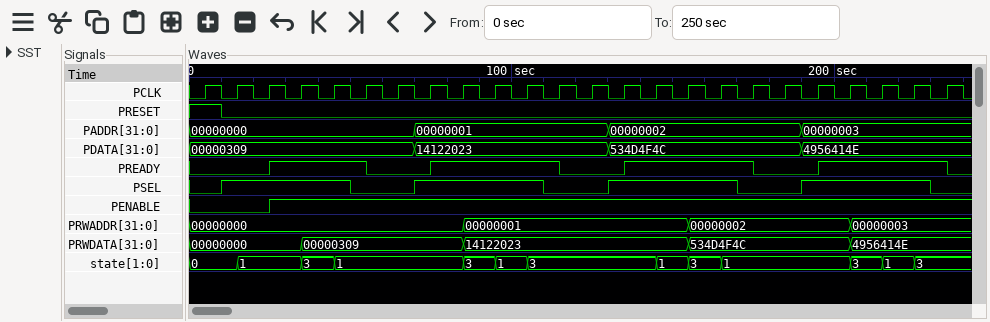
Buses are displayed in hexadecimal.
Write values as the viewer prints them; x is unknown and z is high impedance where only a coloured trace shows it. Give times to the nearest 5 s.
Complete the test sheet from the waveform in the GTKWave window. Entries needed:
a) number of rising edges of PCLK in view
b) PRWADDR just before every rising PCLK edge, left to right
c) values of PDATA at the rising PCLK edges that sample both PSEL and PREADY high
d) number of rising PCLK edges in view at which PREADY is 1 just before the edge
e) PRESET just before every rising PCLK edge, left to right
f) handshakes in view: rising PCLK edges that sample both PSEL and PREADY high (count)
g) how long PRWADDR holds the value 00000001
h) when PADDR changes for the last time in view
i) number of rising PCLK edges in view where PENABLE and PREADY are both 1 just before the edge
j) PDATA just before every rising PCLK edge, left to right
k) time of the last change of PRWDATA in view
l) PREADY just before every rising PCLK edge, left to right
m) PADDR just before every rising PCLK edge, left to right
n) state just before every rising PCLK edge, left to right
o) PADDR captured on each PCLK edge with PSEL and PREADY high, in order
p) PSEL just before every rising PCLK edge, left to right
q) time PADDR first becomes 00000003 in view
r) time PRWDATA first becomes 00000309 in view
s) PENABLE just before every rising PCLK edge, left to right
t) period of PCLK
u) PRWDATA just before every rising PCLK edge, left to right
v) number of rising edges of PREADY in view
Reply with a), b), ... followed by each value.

a) 24
b) 00000000, 00000000, 00000000, 00000000, 00000000, 00000000, 00000000, 00000000, 00000000, 00000001, 00000001, 00000001, 00000001, 00000001, 00000001, 00000001, 00000002, 00000002, 00000002, 00000002, 00000002, 00000003, 00000003, 00000003
c) 00000309, 00000309, 14122023, 14122023, 14122023, 534D4F4C, 534D4F4C, 534D4F4C, 4956414E, 4956414E, 4956414E
d) 15
e) 1 0 0 0 0 0 0 0 0 0 0 0 0 0 0 0 0 0 0 0 0 0 0 0
f) 11
g) 70 s
h) 190 s
i) 15
j) 00000309, 00000309, 00000309, 00000309, 00000309, 00000309, 00000309, 14122023, 14122023, 14122023, 14122023, 14122023, 14122023, 534D4F4C, 534D4F4C, 534D4F4C, 534D4F4C, 534D4F4C, 534D4F4C, 4956414E, 4956414E, 4956414E, 4956414E, 4956414E
k) 205 s
l) 0 0 0 1 1 1 0 0 1 1 1 1 0 0 1 1 1 1 0 0 1 1 1 1
m) 00000000, 00000000, 00000000, 00000000, 00000000, 00000000, 00000000, 00000001, 00000001, 00000001, 00000001, 00000001, 00000001, 00000002, 00000002, 00000002, 00000002, 00000002, 00000002, 00000003, 00000003, 00000003, 00000003, 00000003
n) 0, 0, 1, 1, 3, 1, 1, 1, 1, 3, 1, 3, 3, 3, 3, 1, 3, 1, 1, 1, 1, 3, 1, 3
o) 00000000, 00000000, 00000001, 00000001, 00000001, 00000002, 00000002, 00000002, 00000003, 00000003, 00000003
p) 0 1 1 1 1 0 0 1 1 1 1 0 0 1 1 1 1 0 0 1 1 1 1 0
q) 190 s
r) 35 s
s) 0 0 0 1 1 1 1 1 1 1 1 1 1 1 1 1 1 1 1 1 1 1 1 1
t) 10 s
u) 00000000, 00000000, 00000000, 00000000, 00000309, 00000309, 00000309, 00000309, 00000309, 14122023, 14122023, 14122023, 14122023, 14122023, 14122023, 14122023, 534D4F4C, 534D4F4C, 534D4F4C, 534D4F4C, 534D4F4C, 4956414E, 4956414E, 4956414E
v) 4
